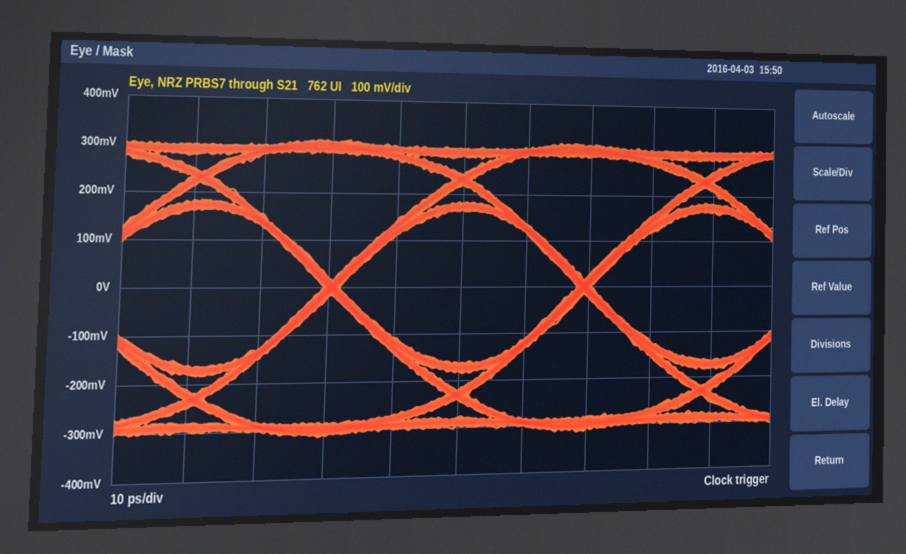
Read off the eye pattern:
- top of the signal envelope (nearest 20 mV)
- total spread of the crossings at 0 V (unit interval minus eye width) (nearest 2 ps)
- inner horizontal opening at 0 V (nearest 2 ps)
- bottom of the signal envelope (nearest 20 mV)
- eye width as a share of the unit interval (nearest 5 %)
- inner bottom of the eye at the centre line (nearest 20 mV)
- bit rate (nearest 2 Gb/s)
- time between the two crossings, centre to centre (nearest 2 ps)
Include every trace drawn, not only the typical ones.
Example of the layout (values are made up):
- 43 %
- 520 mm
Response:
- 320 mV
- 2 ps
- 36 ps
- -320 mV
- 95 %
- -160 mV
- 26 Gb/s
- 38 ps
